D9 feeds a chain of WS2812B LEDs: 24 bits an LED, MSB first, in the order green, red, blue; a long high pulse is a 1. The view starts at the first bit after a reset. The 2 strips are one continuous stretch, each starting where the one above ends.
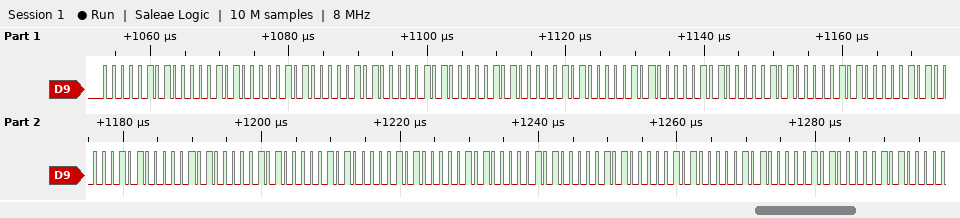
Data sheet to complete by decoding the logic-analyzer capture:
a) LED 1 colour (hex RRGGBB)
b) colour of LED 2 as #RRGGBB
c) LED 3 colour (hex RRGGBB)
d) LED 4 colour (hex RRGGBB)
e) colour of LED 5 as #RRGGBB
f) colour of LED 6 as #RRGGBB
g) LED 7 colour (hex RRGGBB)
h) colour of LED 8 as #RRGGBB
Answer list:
#050505
#050505
#050505
#050505
#050505
#050505
#050505
#050505
